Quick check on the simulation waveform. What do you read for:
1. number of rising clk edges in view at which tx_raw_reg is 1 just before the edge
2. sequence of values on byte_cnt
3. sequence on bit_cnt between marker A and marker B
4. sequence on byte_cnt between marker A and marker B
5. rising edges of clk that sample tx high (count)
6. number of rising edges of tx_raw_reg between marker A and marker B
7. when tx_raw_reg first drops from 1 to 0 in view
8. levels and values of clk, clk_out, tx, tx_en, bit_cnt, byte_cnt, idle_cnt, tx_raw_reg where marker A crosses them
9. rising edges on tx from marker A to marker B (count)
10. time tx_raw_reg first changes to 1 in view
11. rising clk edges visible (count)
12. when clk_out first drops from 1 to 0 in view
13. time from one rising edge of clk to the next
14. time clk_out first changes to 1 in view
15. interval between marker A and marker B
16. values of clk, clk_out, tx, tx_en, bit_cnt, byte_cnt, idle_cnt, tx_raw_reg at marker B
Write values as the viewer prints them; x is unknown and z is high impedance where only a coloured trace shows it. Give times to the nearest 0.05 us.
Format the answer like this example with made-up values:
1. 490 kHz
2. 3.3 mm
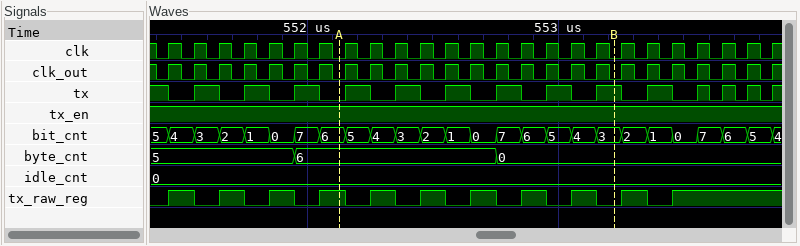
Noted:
1. 14
2. 5, 6, 0
3. 6, 5, 4, 3, 2, 1, 0, 7, 6, 5, 4, 3
4. 6, 0
5. 11
6. 5
7. 551.55 us
8. clk=0, clk_out=0, tx=0, tx_en=1, bit_cnt=6, byte_cnt=6, idle_cnt=0, tx_raw_reg=1
9. 6
10. 551.45 us
11. 25
12. 551.4 us
13. 0.1 us
14. 551.45 us
15. 1.1 us
16. clk=0, clk_out=0, tx=1, tx_en=1, bit_cnt=3, byte_cnt=0, idle_cnt=0, tx_raw_reg=0
